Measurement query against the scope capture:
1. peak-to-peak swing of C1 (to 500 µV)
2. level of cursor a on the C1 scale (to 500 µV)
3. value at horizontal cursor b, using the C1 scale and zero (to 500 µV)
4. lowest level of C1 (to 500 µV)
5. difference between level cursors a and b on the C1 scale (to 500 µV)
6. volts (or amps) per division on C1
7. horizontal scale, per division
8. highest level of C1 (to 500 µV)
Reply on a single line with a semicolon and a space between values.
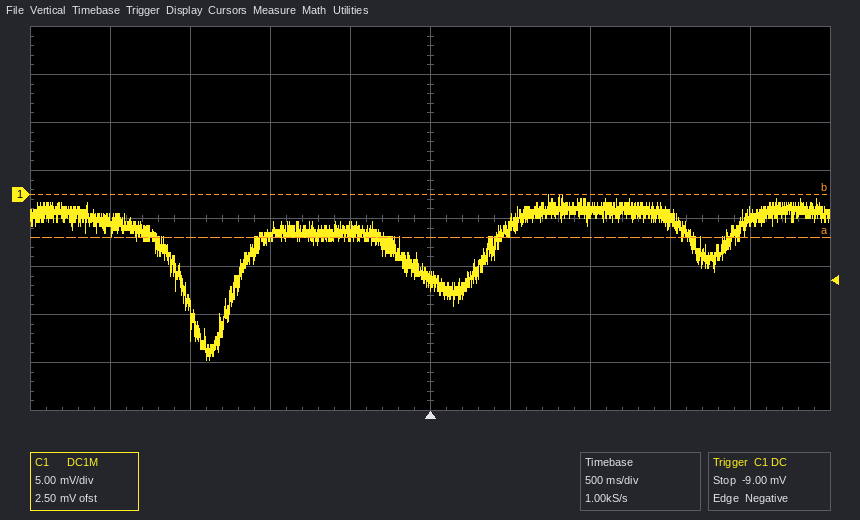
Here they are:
17.0 mV; -4.5 mV; 0.0 mV; -17.0 mV; 4.5 mV; 5 mV; 500 ms; 0.0 mV
